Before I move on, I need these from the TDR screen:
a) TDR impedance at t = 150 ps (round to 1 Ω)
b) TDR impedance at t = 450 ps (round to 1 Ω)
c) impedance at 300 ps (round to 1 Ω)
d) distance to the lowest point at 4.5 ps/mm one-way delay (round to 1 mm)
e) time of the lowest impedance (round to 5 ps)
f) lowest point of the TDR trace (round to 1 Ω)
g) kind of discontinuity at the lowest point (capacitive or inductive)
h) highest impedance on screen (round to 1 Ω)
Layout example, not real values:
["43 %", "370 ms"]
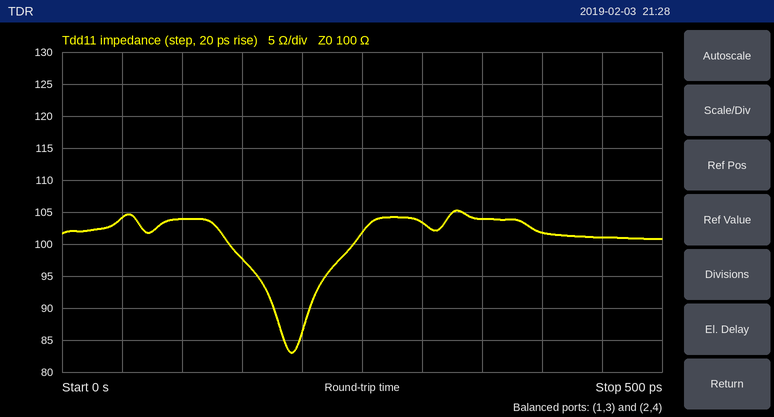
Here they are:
["98 Ω", "101 Ω", "103 Ω", "21 mm", "190 ps", "83 Ω", "capacitive", "105 Ω"]
